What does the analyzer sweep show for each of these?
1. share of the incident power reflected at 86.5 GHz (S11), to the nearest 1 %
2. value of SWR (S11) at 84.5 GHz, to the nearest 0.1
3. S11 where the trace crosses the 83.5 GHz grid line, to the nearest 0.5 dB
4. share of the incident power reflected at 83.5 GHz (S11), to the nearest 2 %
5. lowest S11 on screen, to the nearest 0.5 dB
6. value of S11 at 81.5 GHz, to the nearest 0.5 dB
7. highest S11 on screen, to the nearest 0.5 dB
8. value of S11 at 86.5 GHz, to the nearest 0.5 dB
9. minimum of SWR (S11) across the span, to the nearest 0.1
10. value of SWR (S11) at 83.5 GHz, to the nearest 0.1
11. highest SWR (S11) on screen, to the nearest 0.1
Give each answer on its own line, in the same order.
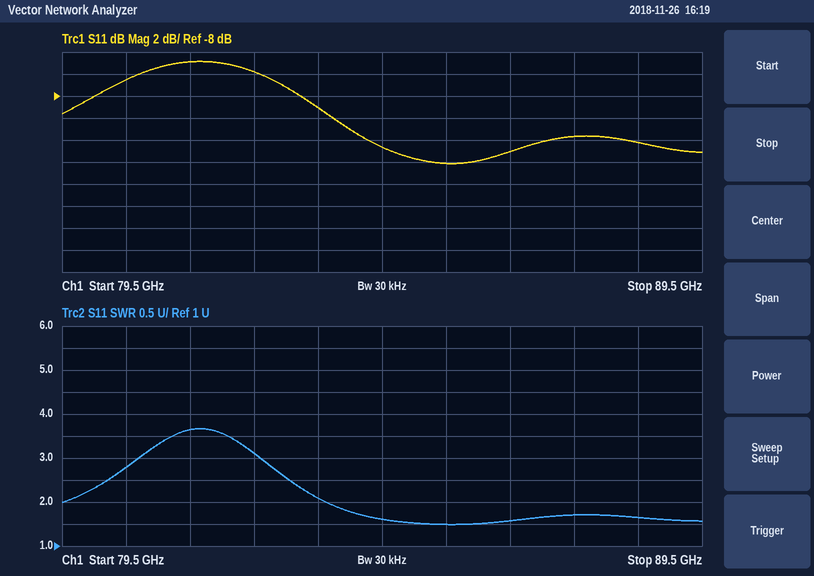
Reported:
5 %
1.6
-9.0 dB
12 %
-14.0 dB
-5.0 dB
-5.0 dB
-13.0 dB
1.5
2.1
3.7
